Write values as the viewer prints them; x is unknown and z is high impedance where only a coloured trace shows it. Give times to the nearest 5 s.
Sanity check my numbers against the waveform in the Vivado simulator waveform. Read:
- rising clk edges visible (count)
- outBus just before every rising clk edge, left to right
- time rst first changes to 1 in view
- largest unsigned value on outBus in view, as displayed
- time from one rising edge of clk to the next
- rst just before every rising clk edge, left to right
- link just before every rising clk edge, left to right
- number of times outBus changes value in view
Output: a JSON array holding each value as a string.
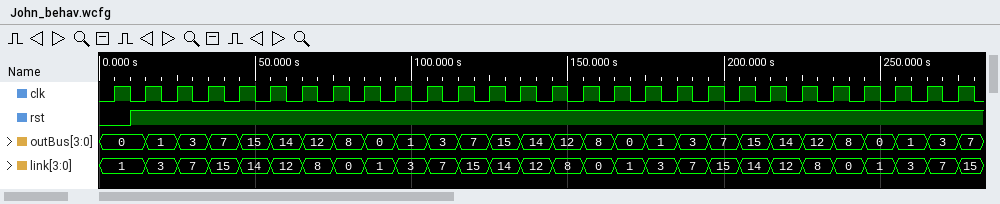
["28", "0, 0, 1, 3, 7, 15, 14, 12, 8, 0, 1, 3, 7, 15, 14, 12, 8, 0, 1, 3, 7, 15, 14, 12, 8, 0, 1, 3", "10 s", "15", "10 s", "0 1 1 1 1 1 1 1 1 1 1 1 1 1 1 1 1 1 1 1 1 1 1 1 1 1 1 1", "1, 1, 3, 7, 15, 14, 12, 8, 0, 1, 3, 7, 15, 14, 12, 8, 0, 1, 3, 7, 15, 14, 12, 8, 0, 1, 3, 7", "27"]
